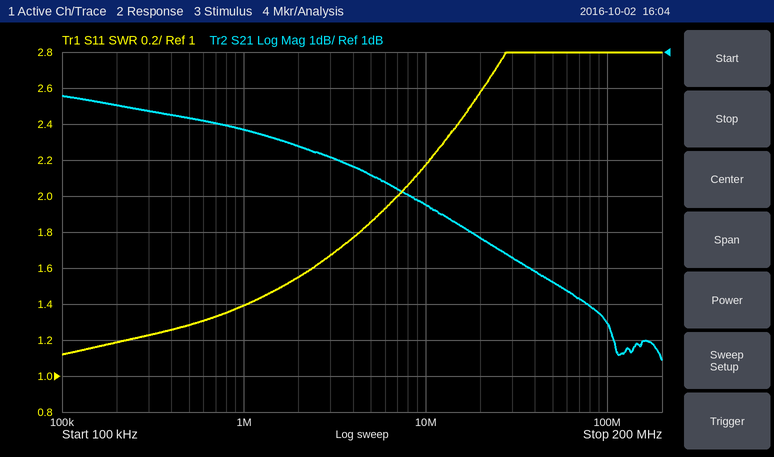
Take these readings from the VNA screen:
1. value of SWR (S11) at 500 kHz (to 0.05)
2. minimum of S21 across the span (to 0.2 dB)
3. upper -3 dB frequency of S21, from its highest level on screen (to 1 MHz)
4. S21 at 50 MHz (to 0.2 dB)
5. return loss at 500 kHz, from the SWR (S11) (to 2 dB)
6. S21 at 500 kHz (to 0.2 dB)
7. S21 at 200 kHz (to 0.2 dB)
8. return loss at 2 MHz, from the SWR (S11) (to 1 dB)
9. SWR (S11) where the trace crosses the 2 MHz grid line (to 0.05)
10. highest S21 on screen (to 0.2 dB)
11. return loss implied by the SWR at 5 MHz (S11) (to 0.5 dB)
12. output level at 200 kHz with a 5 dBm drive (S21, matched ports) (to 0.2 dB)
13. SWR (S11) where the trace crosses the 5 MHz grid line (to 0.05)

1.30
-7.6 dB
10 MHz
-5.4 dB
18 dB
-0.8 dB
-0.4 dB
13 dB
1.55
-0.2 dB
10.5 dB
4.6 dBm
1.85
